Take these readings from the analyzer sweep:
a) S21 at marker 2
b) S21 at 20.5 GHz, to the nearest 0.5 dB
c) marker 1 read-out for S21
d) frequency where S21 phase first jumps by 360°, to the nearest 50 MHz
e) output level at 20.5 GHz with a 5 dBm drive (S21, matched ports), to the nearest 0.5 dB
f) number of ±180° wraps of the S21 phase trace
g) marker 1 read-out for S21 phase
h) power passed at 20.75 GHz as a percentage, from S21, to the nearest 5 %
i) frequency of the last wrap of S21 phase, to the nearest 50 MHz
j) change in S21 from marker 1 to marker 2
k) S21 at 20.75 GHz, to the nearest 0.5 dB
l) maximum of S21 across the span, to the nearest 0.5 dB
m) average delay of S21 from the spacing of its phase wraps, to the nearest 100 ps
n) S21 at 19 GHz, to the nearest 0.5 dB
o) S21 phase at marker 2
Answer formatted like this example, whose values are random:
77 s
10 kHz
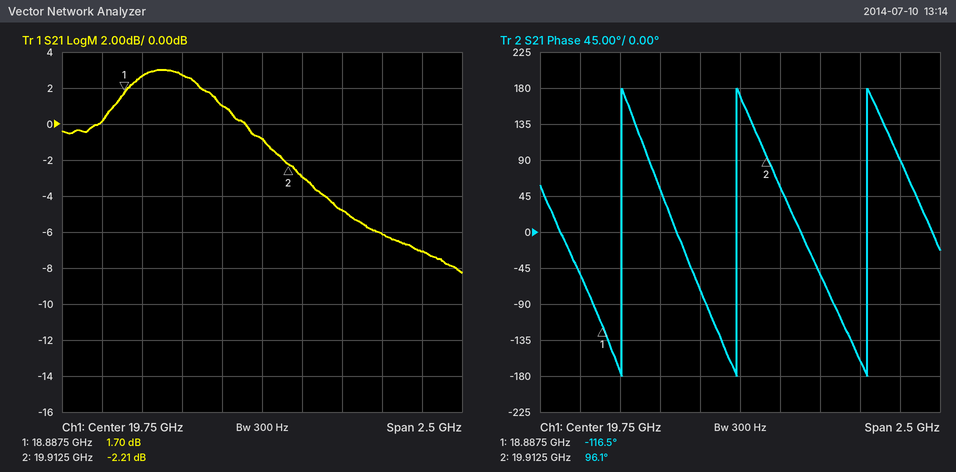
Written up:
-2.21 dB
-6.0 dB
1.70 dB
19.00 GHz
-1.0 dBm
3
-116.5°
20 %
20.55 GHz
-3.91 dB
-7.0 dB
3.0 dB
1.3 ns
2.5 dB
96.1°
